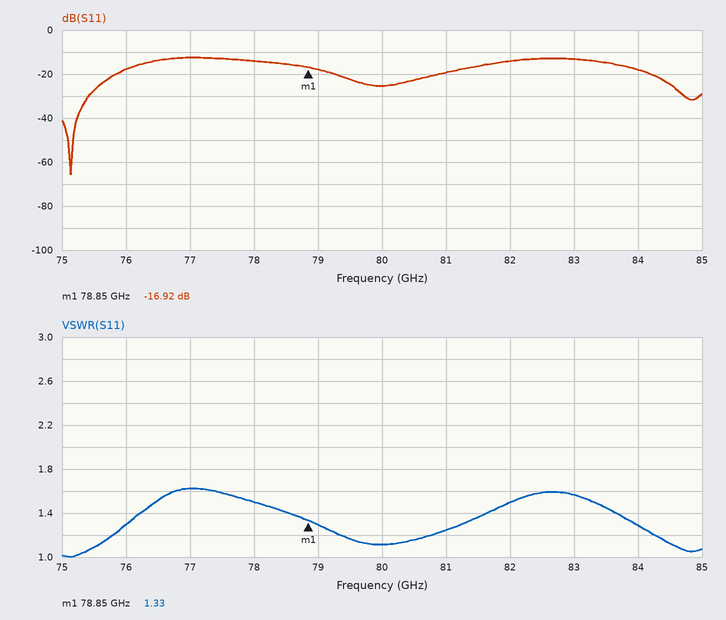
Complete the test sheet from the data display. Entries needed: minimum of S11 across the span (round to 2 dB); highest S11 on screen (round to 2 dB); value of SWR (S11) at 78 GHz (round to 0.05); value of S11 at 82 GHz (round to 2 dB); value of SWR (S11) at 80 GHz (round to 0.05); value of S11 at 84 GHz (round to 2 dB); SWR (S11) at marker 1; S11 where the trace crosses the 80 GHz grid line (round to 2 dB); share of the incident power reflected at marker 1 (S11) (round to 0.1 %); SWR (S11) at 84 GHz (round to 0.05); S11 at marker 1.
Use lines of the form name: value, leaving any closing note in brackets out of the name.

minimum of S11 across the span: -66 dB
highest S11 on screen: -12 dB
value of SWR (S11) at 78 GHz: 1.50
value of S11 at 82 GHz: -14 dB
value of SWR (S11) at 80 GHz: 1.10
value of S11 at 84 GHz: -18 dB
SWR (S11) at marker 1: 1.33
S11 where the trace crosses the 80 GHz grid line: -26 dB
share of the incident power reflected at marker 1 (S11): 2.0 %
SWR (S11) at 84 GHz: 1.30
S11 at marker 1: -16.92 dB
